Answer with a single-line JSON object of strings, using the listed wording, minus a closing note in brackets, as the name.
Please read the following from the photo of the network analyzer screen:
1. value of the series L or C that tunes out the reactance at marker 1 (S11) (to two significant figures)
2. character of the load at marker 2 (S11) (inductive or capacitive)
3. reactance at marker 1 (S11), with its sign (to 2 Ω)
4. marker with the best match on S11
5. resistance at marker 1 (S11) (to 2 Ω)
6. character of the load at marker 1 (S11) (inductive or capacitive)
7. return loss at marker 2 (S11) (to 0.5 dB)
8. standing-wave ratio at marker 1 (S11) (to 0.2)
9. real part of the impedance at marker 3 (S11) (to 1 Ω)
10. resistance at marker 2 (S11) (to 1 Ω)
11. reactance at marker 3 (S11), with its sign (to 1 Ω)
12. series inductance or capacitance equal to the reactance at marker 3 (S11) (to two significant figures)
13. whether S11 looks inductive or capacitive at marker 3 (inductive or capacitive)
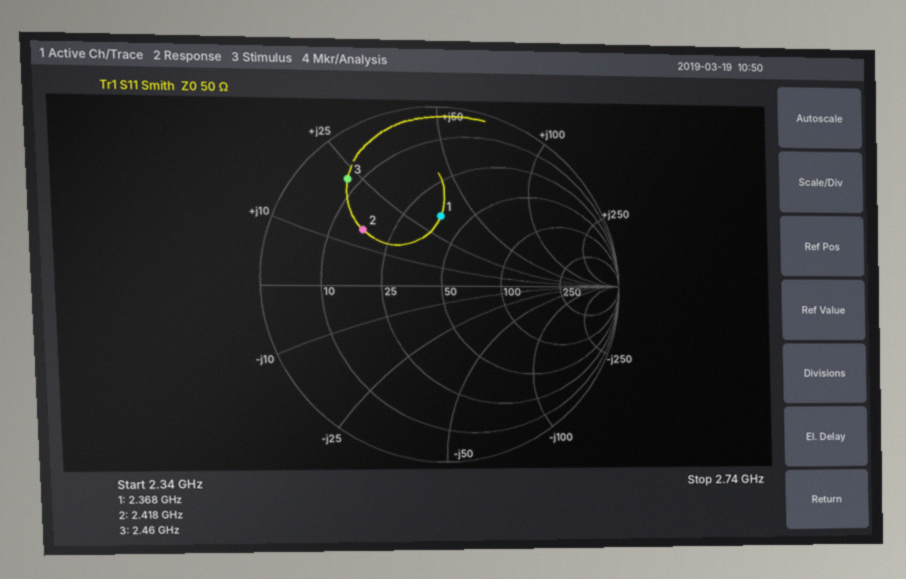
{"value of the series L or C that tunes out the reactance at marker 1 (S11)": "2.0 pF", "character of the load at marker 2 (S11)": "inductive", "reactance at marker 1 (S11), with its sign": "+34 Ω", "marker with the best match on S11": "marker 1", "resistance at marker 1 (S11)": "38 Ω", "character of the load at marker 1 (S11)": "inductive", "return loss at marker 2 (S11)": "5.5 dB", "standing-wave ratio at marker 1 (S11)": "2.2", "real part of the impedance at marker 3 (S11)": "8 Ω", "resistance at marker 2 (S11)": "17 Ω", "reactance at marker 3 (S11), with its sign": "+23 Ω", "series inductance or capacitance equal to the reactance at marker 3 (S11)": "1.5 nH", "whether S11 looks inductive or capacitive at marker 3": "inductive"}
